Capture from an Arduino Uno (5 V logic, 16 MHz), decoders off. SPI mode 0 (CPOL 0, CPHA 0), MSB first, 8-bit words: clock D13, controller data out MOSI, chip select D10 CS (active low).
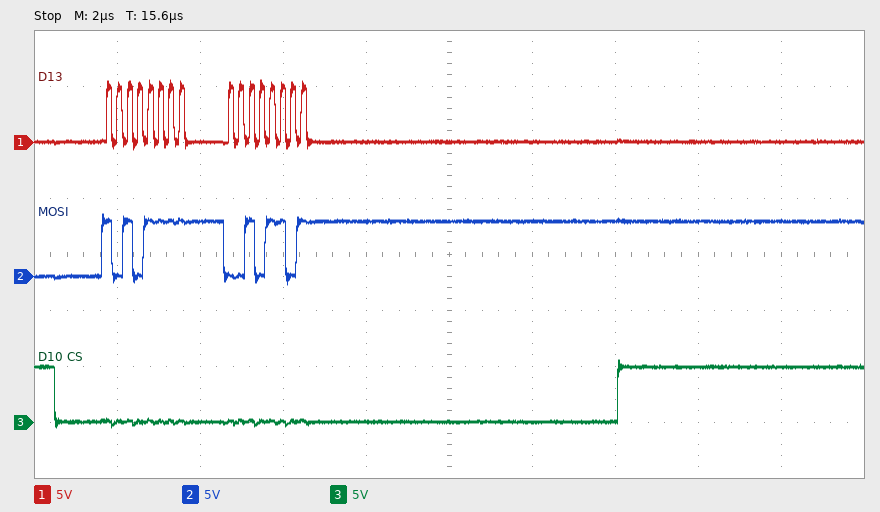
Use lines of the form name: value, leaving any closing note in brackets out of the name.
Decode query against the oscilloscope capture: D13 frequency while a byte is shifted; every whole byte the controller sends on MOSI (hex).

D13 frequency while a byte is shifted: 4 MHz
every whole byte the controller sends on MOSI: AF 2D
